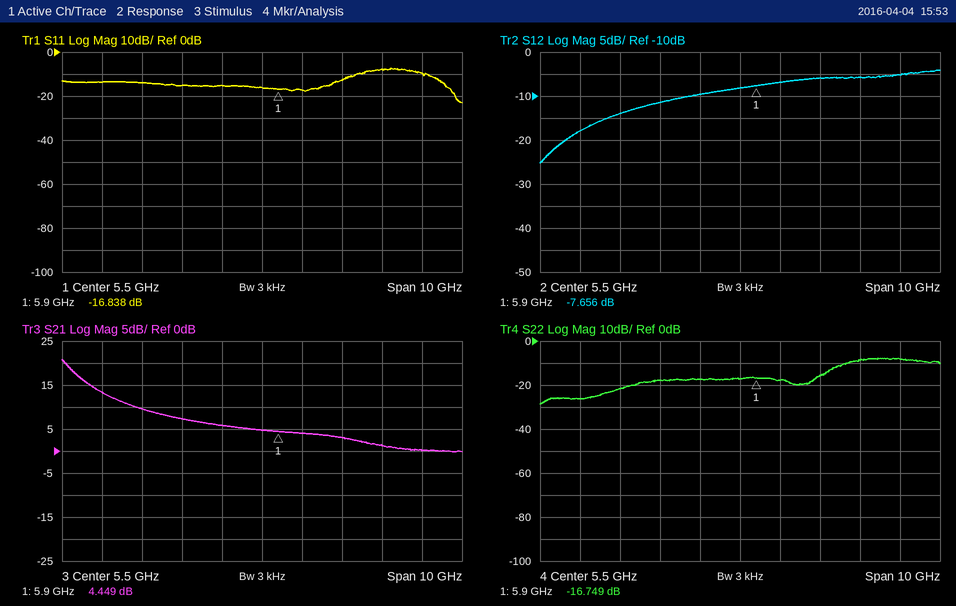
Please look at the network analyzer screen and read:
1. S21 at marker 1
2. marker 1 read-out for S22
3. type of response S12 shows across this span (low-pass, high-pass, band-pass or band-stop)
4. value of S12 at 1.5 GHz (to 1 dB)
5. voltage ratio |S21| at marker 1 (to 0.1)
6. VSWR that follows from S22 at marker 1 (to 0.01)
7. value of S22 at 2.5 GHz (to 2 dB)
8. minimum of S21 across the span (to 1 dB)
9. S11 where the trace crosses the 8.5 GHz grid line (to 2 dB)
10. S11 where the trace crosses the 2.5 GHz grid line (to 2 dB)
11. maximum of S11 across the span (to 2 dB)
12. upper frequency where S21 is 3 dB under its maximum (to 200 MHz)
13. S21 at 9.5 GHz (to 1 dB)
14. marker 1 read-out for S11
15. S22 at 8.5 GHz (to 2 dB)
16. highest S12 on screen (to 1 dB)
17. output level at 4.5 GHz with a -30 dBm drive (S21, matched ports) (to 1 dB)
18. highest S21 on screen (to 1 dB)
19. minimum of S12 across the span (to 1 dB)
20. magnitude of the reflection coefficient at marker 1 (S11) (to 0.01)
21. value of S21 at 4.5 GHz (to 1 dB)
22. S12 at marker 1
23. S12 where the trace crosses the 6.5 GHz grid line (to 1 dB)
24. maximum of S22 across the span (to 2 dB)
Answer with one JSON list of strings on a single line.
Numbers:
["4.449 dB", "-16.749 dB", "high-pass", "-18 dB", "1.7", "1.34", "-22 dB", "0 dB", "-8 dB", "-14 dB", "-8 dB", "800 MHz", "0 dB", "-16.838 dB", "-8 dB", "-4 dB", "-24 dBm", "21 dB", "-25 dB", "0.14", "6 dB", "-7.656 dB", "-7 dB", "-8 dB"]
